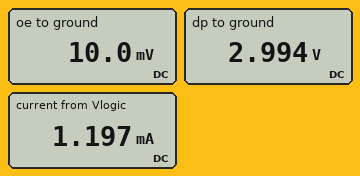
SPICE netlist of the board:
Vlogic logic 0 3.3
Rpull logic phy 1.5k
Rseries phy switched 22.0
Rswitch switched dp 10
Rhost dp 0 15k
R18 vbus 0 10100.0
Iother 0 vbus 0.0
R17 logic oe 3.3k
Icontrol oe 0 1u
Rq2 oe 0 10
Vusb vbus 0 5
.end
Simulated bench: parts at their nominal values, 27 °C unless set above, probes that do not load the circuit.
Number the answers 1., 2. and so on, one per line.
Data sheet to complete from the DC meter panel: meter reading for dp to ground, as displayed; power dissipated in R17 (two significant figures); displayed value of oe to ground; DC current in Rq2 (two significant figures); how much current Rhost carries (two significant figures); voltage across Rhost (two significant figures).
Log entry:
1. 2.994 V
2. 3.3 mW
3. 10.0 mV
4. 1.0 mA
5. 200 µA
6. 3.0 V
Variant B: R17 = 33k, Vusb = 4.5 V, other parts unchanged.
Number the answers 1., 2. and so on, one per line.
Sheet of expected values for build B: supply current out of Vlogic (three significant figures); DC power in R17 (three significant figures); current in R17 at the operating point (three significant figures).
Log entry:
1. 300 µA
2. 330 µW
3. 100 µA
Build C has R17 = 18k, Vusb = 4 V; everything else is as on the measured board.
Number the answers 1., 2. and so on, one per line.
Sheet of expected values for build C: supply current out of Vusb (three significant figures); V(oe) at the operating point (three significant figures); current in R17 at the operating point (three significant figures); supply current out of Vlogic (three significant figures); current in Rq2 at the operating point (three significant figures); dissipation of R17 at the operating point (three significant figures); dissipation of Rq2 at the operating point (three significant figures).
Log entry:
1. 396 µA
2. 1.82 mV
3. 183 µA
4. 383 µA
5. 182 µA
6. 604 µW
7. 332 nW
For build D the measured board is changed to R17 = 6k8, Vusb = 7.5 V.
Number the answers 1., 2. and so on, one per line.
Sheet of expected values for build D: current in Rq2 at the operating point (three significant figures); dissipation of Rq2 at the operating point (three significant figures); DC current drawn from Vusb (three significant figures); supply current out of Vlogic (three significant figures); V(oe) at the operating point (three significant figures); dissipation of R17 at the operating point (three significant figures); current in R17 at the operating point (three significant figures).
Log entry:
1. 484 µA
2. 2.34 µW
3. 743 µA
4. 684 µA
5. 4.84 mV
6. 1.60 mW
7. 485 µA
